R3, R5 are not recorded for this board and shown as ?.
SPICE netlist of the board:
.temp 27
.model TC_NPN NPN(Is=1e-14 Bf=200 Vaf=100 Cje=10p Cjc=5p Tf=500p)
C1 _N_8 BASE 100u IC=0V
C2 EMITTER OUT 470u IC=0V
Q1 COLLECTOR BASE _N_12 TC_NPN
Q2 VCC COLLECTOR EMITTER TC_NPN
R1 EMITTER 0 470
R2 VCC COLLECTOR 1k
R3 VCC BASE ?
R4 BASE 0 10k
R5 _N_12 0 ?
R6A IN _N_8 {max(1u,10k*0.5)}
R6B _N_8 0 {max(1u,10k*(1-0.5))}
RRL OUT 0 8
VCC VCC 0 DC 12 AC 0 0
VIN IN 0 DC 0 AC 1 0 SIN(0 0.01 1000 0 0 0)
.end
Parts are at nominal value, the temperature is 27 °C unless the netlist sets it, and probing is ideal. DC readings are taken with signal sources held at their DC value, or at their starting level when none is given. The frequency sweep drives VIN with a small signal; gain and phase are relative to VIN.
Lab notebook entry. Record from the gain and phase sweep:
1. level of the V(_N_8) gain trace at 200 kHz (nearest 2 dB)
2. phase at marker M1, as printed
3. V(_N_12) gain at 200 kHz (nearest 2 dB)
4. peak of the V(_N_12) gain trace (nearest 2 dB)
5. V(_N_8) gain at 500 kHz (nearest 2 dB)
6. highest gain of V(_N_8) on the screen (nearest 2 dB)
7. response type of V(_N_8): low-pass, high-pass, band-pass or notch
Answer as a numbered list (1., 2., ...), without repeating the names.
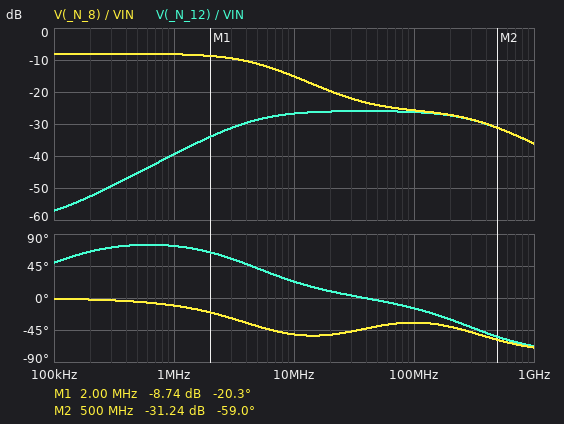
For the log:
1. -8 dB
2. -20.3 deg
3. -52 dB
4. -26 dB
5. -8 dB
6. -8 dB
7. low-pass
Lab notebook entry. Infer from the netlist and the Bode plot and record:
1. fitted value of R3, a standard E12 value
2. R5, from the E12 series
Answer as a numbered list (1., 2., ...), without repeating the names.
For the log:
1. 270 kΩ
2. 330 Ω
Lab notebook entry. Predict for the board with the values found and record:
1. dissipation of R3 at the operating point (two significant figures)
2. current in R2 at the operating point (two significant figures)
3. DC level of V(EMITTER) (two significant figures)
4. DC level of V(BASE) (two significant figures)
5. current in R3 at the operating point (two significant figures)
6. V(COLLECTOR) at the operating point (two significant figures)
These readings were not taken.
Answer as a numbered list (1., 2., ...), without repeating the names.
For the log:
1. 500 µW
2. 120 µA
3. 11 V
4. 430 mV
5. 43 µA
6. 12 V
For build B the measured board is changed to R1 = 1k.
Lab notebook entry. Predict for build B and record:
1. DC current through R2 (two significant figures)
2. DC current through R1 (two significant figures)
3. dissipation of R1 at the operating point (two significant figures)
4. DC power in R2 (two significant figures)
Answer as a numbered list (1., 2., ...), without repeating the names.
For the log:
1. 56 µA
2. 11 mA
3. 130 mW
4. 3.1 µW
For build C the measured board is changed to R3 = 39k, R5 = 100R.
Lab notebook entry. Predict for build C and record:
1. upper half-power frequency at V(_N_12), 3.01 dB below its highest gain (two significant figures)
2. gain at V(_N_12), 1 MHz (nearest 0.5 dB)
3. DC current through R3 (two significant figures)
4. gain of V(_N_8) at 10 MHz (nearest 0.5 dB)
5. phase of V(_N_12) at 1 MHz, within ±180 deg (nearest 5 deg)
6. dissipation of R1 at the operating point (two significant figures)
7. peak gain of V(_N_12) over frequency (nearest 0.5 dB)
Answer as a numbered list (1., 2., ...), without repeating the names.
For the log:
1. 61 MHz
2. -29.5 dB
3. 260 µA
4. -27.0 dB
5. 0 deg
6. 720 µW
7. -25.5 dB
